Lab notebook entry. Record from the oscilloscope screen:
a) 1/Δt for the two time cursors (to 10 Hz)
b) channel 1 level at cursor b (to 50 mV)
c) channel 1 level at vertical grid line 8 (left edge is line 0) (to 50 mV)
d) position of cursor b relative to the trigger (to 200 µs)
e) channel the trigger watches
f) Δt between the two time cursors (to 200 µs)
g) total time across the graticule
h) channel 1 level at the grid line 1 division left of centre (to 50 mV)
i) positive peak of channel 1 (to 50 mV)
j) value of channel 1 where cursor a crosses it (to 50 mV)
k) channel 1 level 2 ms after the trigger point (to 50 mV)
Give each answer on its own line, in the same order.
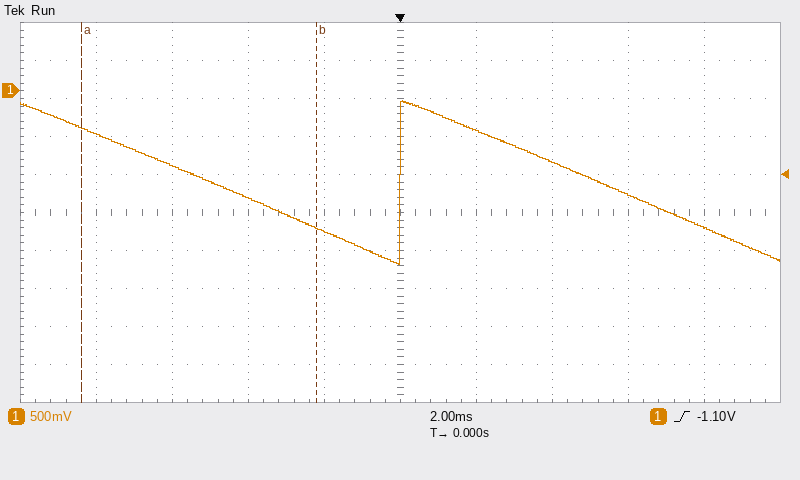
160 Hz
-1.80 V
-1.35 V
-2.2 ms
channel 1
6.2 ms
20 ms
-1.85 V
-150 mV
-500 mV
-500 mV
